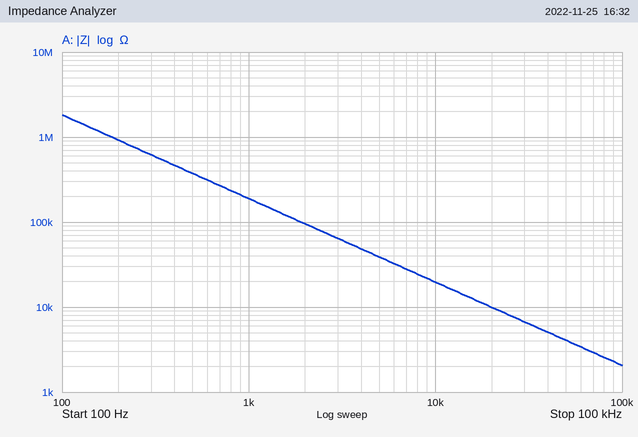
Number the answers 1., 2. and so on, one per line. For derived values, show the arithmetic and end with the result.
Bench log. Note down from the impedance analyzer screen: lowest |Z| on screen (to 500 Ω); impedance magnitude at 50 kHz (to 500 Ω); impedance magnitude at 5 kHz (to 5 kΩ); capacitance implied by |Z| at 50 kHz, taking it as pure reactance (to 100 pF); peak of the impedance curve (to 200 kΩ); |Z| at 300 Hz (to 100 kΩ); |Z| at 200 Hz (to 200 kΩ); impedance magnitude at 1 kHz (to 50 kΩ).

1. 2.0 kΩ
2. 4.0 kΩ
3. 40 kΩ
4. C = 1/(2π × 50 kHz × 4.0 kΩ) ≈ 796 pF, so 800 pF to the nearest 100 pF
5. 1.8 MΩ
6. 600 kΩ
7. 1.0 MΩ
8. 200 kΩ
